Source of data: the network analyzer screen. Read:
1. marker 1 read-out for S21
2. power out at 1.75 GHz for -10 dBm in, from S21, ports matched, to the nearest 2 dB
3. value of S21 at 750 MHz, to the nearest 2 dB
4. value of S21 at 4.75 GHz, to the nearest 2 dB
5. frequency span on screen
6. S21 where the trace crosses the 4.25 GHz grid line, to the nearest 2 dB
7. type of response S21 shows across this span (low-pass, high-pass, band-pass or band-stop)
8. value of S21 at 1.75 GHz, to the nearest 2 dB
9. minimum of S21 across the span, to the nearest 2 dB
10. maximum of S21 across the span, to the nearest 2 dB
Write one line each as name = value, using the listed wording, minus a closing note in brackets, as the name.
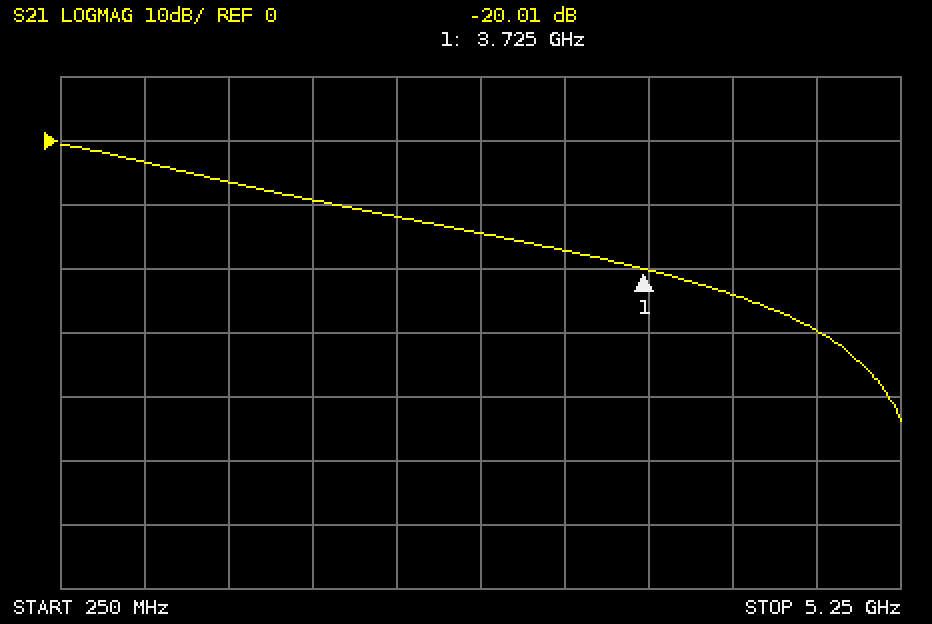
marker 1 read-out for S21 = -20.01 dB
power out at 1.75 GHz for -10 dBm in, from S21, ports matched, to the nearest 2 dB = -20 dBm
value of S21 at 750 MHz, to the nearest 2 dB = -4 dB
value of S21 at 4.75 GHz, to the nearest 2 dB = -30 dB
frequency span on screen = 5 GHz
S21 where the trace crosses the 4.25 GHz grid line, to the nearest 2 dB = -24 dB
type of response S21 shows across this span = low-pass
value of S21 at 1.75 GHz, to the nearest 2 dB = -10 dB
minimum of S21 across the span, to the nearest 2 dB = -44 dB
maximum of S21 across the span, to the nearest 2 dB = 0 dB
